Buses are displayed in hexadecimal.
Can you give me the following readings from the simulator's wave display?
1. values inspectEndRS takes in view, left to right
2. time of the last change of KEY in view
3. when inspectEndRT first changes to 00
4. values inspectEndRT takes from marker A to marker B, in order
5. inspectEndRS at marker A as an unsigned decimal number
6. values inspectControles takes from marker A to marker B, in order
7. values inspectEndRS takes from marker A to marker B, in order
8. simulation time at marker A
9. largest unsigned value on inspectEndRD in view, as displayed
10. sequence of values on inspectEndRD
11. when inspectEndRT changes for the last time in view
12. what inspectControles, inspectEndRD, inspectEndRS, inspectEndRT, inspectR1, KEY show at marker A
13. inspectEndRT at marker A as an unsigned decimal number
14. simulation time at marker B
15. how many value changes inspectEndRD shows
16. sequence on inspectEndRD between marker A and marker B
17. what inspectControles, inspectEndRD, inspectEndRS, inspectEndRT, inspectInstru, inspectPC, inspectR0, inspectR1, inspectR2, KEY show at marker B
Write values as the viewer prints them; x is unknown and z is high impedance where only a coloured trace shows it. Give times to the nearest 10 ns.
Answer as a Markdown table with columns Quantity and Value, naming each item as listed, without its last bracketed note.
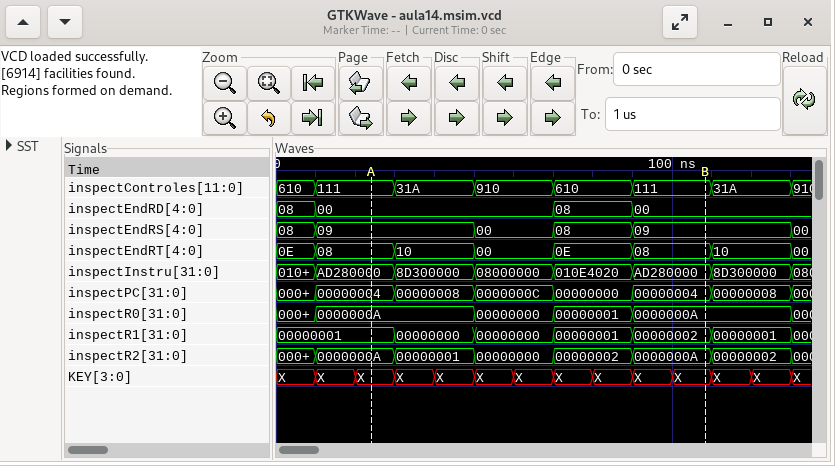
| Quantity | Value |
|---|---|
| values inspectEndRS takes in view, left to right | 08, 09, 00, 08, 09, 00 |
| time of the last change of KEY in view | 130 ns |
| when inspectEndRT first changes to 00 | 50 ns |
| values inspectEndRT takes from marker A to marker B, in order | 08, 10, 00, 0E, 08 |
| inspectEndRS at marker A as an unsigned decimal number | 9 |
| values inspectControles takes from marker A to marker B, in order | 111, 31A, 910, 610, 111 |
| values inspectEndRS takes from marker A to marker B, in order | 09, 00, 08, 09 |
| simulation time at marker A | 20 ns |
| largest unsigned value on inspectEndRD in view, as displayed | 08 |
| sequence of values on inspectEndRD | 08, 00, 08, 00 |
| when inspectEndRT changes for the last time in view | 130 ns |
| what inspectControles, inspectEndRD, inspectEndRS, inspectEndRT, inspectR1, KEY show at marker A | inspectControles=111, inspectEndRD=00, inspectEndRS=09, inspectEndRT=08, inspectR1=00000001, KEY=X |
| inspectEndRT at marker A as an unsigned decimal number | 8 |
| simulation time at marker B | 110 ns |
| how many value changes inspectEndRD shows | 3 |
| sequence on inspectEndRD between marker A and marker B | 00, 08, 00 |
| what inspectControles, inspectEndRD, inspectEndRS, inspectEndRT, inspectInstru, inspectPC, inspectR0, inspectR1, inspectR2, KEY show at marker B | inspectControles=111, inspectEndRD=00, inspectEndRS=09, inspectEndRT=08, inspectInstru=AD280000, inspectPC=00000004, inspectR0=0000000A, inspectR1=00000002, inspectR2=0000000A, KEY=X |
